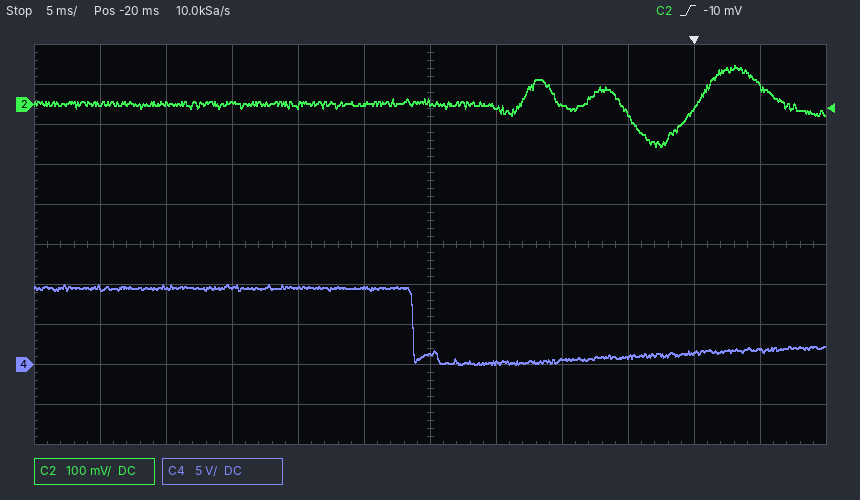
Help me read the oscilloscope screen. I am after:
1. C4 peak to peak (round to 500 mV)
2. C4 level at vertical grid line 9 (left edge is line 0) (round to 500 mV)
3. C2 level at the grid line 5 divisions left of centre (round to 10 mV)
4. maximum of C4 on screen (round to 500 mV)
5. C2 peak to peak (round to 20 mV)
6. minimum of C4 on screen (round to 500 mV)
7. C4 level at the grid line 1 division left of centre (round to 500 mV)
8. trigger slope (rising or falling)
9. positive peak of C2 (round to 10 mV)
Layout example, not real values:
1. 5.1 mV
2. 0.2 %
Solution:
1. 10.0 V
2. 1.0 V
3. 0 mV
4. 10.0 V
5. 200 mV
6. 0.0 V
7. 9.5 V
8. rising
9. 100 mV
